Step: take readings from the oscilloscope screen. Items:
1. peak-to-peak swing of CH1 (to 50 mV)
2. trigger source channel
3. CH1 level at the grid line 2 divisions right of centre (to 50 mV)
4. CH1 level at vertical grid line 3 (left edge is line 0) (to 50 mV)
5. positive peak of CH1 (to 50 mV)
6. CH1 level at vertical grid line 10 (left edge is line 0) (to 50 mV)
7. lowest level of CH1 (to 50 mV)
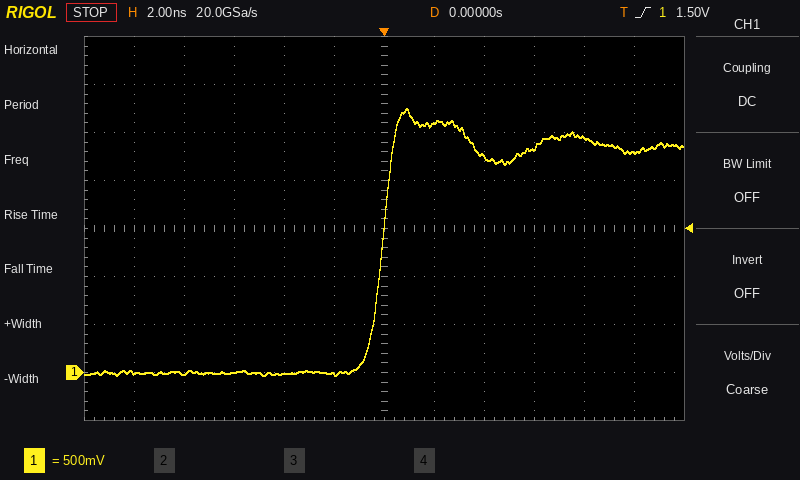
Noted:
2.80 V
CH1
2.25 V
0 mV
2.75 V
2.45 V
-50 mV
